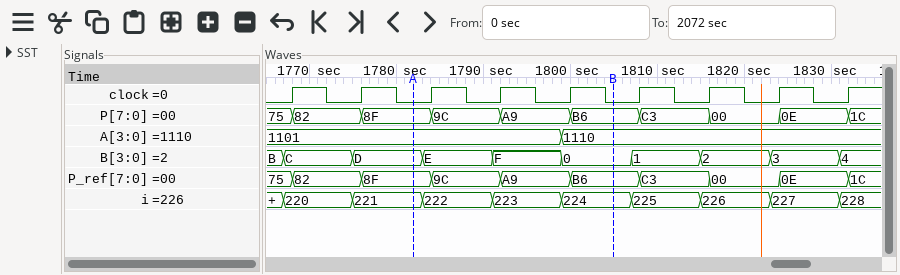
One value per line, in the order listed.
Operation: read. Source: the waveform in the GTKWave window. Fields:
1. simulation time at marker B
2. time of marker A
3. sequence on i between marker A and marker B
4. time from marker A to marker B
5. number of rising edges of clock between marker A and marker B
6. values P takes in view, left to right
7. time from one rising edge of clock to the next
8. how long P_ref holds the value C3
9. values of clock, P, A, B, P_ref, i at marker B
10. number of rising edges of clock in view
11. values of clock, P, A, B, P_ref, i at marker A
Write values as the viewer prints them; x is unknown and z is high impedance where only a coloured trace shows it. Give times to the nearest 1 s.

1805 s
1782 s
221, 222, 223, 224
23 s
3
75, 82, 8F, 9C, A9, B6, C3, 00, 0E, 1C
8 s
8 s
clock=0, P=B6, A=1110, B=0, P_ref=B6, i=224
9
clock=0, P=8F, A=1101, B=D, P_ref=8F, i=221
